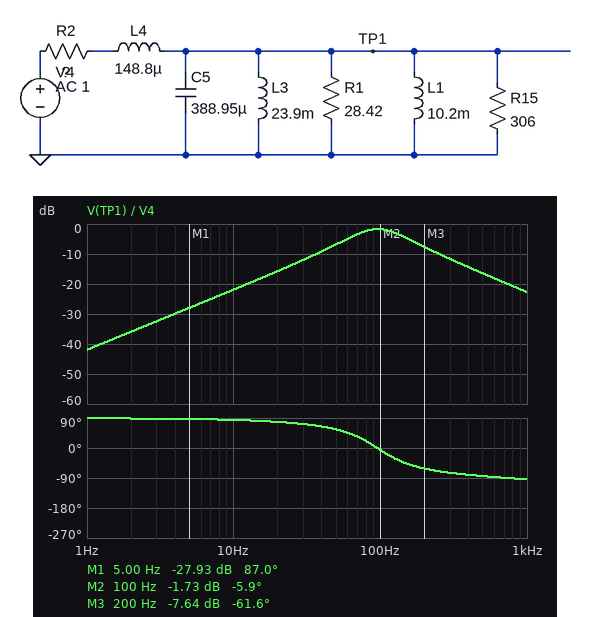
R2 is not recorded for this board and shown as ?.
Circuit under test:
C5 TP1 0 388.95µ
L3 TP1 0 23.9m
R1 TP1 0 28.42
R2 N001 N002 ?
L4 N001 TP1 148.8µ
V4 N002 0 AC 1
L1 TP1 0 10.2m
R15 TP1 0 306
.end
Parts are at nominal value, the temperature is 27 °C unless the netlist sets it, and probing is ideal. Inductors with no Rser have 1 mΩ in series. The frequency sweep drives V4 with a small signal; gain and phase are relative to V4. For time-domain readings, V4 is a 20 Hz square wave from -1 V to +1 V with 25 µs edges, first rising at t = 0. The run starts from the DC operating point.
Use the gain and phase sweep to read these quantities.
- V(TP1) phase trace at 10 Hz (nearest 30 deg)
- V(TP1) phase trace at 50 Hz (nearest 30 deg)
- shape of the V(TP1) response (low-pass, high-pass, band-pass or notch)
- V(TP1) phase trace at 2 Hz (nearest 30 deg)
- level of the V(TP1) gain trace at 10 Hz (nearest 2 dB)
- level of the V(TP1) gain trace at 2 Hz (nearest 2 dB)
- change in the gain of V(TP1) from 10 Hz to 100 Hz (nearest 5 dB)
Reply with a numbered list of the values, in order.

1. 90 deg
2. 60 deg
3. band-pass
4. 90 deg
5. -22 dB
6. -36 dB
7. 20 dB
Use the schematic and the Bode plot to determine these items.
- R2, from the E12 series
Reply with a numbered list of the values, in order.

1. 5.6 Ω
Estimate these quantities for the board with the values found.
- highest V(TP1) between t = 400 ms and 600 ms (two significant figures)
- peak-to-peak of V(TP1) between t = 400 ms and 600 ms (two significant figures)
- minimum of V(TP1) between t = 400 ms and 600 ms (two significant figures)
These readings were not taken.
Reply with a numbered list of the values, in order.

1. 870 mV
2. 1.7 V
3. -870 mV
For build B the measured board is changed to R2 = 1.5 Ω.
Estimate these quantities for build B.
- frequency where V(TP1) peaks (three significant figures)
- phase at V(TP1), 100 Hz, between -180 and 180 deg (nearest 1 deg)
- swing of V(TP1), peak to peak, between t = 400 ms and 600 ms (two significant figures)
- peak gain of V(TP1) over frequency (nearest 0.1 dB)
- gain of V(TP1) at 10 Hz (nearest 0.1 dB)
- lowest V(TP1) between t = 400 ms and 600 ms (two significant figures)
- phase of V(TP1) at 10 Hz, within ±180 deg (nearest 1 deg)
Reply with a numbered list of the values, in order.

1. 106 Hz
2. -2 deg
3. 3.2 V
4. -0.5 dB
5. -10.8 dB
6. -1.6 V
7. 72 deg
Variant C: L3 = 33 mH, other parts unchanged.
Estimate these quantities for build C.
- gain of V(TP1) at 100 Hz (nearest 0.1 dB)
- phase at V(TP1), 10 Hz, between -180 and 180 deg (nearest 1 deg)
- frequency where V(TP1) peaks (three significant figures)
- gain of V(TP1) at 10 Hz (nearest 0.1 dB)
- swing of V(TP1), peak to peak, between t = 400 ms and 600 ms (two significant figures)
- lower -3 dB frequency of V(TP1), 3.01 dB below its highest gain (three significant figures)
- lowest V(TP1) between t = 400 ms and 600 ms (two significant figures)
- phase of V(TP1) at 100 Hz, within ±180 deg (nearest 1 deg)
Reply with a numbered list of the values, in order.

1. -1.8 dB
2. 84 deg
3. 92.0 Hz
4. -21.1 dB
5. 1.8 V
6. 57.4 Hz
7. -890 mV
8. -11 deg
